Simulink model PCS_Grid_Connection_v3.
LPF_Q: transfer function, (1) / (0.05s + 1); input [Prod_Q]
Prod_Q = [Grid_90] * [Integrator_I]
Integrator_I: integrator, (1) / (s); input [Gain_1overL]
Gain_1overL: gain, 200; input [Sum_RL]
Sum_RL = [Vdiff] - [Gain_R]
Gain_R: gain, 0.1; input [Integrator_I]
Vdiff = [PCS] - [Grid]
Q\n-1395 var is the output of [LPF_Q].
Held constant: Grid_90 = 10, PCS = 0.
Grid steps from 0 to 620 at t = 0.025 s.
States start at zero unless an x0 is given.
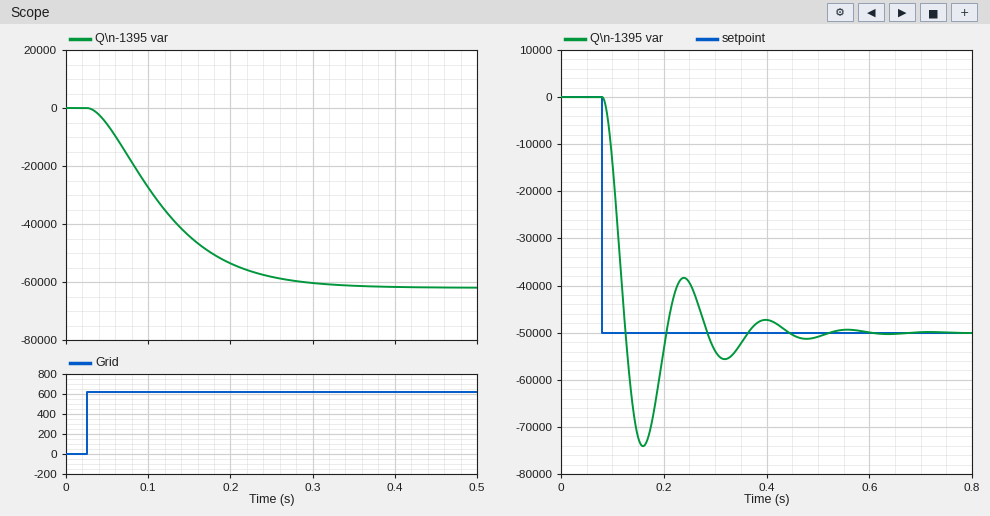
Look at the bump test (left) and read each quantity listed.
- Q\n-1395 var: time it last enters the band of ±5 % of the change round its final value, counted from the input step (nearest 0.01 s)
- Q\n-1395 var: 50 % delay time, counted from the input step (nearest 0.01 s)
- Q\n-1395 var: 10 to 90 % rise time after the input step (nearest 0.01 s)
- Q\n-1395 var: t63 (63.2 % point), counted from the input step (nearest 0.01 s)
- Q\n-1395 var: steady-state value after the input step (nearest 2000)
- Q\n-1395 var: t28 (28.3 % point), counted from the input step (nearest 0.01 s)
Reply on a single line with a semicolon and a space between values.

0.24 s; 0.08 s; 0.17 s; 0.11 s; -62000; 0.05 s
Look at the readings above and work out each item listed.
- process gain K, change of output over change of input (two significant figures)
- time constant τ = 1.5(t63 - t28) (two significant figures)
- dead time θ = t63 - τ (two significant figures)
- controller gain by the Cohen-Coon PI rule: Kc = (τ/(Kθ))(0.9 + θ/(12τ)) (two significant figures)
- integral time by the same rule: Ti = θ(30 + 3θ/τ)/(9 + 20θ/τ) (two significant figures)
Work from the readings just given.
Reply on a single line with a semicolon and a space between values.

-100; 0.090 s; 0.020 s; -0.041; 0.046 s
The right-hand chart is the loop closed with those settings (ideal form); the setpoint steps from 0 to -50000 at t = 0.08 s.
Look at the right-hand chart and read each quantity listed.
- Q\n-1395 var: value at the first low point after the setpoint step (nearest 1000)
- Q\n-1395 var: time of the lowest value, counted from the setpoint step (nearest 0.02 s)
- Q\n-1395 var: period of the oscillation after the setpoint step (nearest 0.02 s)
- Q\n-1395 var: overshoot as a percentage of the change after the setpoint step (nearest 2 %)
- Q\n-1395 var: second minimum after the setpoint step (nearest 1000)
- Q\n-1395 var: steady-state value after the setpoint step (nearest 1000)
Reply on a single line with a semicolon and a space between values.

-74000; 0.08 s; 0.16 s; 48 %; -56000; -50000
